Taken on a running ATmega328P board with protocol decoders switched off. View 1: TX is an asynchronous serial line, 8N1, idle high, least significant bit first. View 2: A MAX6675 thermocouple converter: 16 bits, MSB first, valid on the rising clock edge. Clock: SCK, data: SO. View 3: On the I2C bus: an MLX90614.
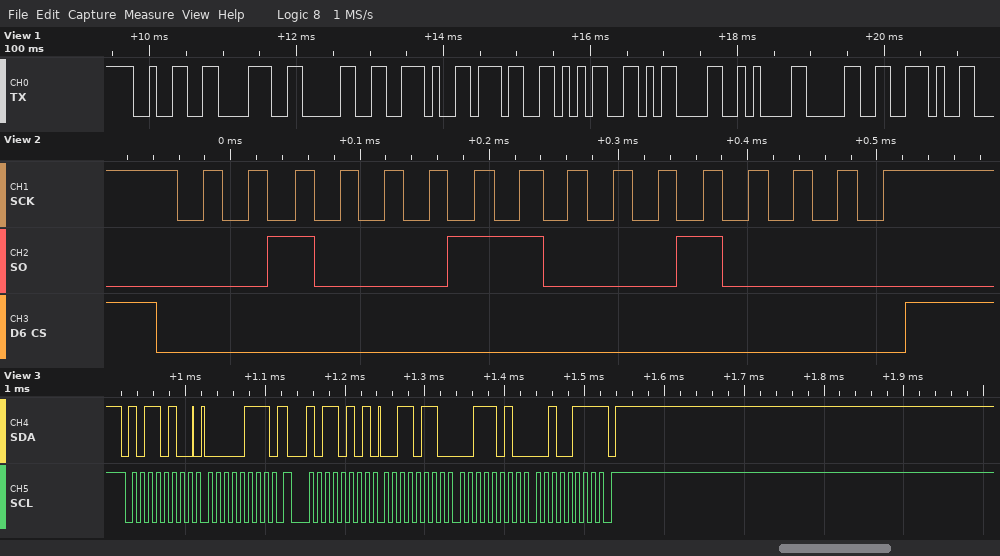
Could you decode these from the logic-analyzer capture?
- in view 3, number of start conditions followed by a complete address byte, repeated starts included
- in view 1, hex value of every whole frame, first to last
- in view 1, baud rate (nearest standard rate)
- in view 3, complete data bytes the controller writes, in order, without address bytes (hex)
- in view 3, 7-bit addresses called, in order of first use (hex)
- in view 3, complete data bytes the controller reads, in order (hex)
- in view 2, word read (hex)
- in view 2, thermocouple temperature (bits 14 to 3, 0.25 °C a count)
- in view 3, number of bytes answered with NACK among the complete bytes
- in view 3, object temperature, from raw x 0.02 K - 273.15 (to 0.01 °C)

2
32 38 30 2E 37 35 0D 0A 30 2E
9600 baud
07
0x5A
36 3A 27
0x2310
280.50 °C
1
24.89 °C
